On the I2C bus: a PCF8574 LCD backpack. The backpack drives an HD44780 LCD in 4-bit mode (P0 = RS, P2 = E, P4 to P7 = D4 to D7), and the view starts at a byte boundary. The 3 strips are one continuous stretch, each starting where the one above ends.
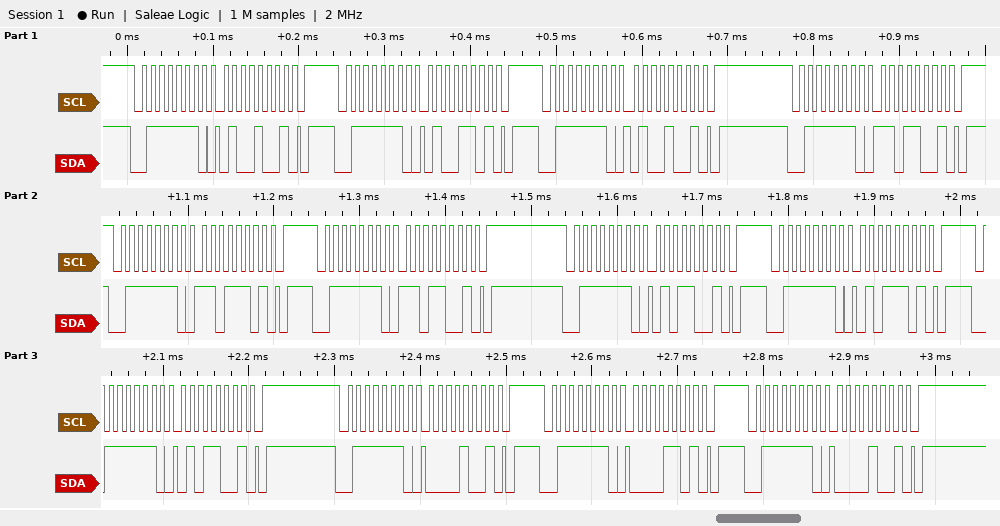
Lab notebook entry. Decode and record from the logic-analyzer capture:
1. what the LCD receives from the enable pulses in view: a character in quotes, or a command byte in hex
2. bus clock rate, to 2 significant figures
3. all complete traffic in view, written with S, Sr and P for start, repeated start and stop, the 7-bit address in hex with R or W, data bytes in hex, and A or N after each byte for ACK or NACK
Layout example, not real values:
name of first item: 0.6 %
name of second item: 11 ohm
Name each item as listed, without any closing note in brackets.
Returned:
what the LCD receives from the enable pulses in view: a character in quotes, or a command byte in hex: 'M' 'P'
bus clock rate, to 2 significant figures: 100 kHz
all complete traffic in view, written with S, Sr and P for start, repeated start and stop, the 7-bit address in hex with R or W, data bytes in hex, and A or N after each byte for ACK or NACK: S 3FW A 49 A P S 3FW A 4D A P S 3FW A 49 A P S 3FW A D9 A P S 3FW A DD A P S 3FW A D9 A P S 3FW A 59 A P S 3FW A 5D A P S 3FW A 59 A P S 3FW A 09 A P S 3FW A 0D A P S 3FW A 09 A P
